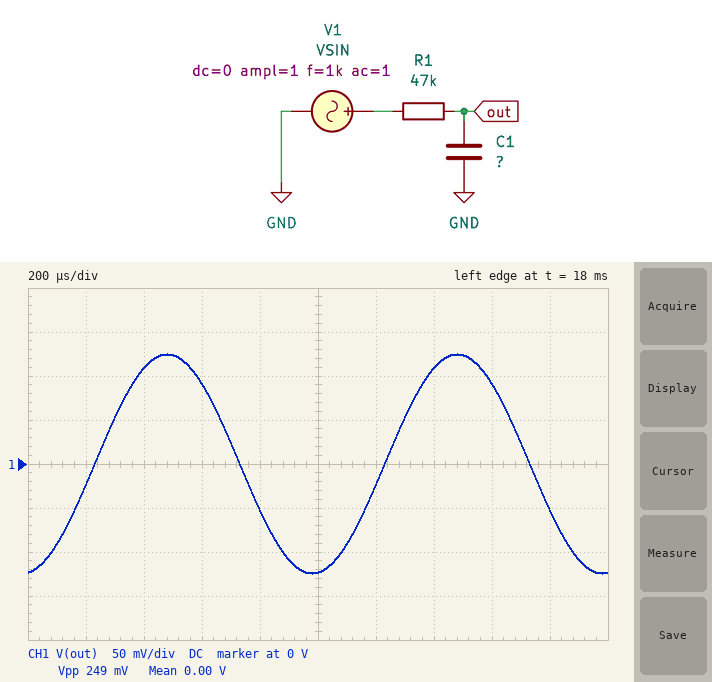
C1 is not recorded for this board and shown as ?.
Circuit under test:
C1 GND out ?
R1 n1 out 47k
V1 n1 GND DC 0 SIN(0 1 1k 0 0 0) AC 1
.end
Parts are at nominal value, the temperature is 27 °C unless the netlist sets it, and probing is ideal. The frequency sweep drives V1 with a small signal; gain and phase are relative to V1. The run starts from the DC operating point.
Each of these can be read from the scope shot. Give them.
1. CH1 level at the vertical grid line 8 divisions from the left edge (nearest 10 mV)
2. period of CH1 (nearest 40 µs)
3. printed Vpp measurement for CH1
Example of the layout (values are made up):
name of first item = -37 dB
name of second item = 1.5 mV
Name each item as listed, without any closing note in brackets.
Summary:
CH1 level at the vertical grid line 8 divisions from the left edge = 90 mV
period of CH1 = 1.00 ms
printed Vpp measurement for CH1 = 249 mV
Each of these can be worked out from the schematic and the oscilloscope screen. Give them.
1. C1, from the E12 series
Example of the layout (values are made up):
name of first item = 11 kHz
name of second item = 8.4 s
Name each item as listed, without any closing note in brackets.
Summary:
C1, from the E12 series = 27 nF
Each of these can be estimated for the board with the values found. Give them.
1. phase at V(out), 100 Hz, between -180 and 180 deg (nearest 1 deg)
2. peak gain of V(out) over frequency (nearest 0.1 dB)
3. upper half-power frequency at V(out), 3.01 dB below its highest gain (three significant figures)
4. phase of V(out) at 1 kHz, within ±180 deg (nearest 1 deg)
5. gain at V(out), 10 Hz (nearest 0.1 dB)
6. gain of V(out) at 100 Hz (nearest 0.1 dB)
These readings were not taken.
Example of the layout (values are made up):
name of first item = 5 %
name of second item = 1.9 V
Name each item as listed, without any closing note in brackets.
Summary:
phase at V(out), 100 Hz, between -180 and 180 deg = -39 deg
peak gain of V(out) over frequency = 0 dB
upper half-power frequency at V(out), 3.01 dB below its highest gain = 125 Hz
phase of V(out) at 1 kHz, within ±180 deg = -83 deg
gain at V(out), 10 Hz = 0 dB
gain of V(out) at 100 Hz = -2.1 dB
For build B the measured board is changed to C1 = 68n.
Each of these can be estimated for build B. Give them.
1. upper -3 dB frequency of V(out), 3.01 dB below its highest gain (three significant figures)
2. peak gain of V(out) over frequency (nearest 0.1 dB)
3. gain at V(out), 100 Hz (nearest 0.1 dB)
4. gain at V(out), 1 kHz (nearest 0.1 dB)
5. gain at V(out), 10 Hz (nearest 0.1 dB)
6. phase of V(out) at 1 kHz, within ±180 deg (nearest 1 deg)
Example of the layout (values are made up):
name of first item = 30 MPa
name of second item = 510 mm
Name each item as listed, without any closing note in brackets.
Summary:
upper -3 dB frequency of V(out), 3.01 dB below its highest gain = 49.8 Hz
peak gain of V(out) over frequency = 0 dB
gain at V(out), 100 Hz = -7.0 dB
gain at V(out), 1 kHz = -26.1 dB
gain at V(out), 10 Hz = -0.2 dB
phase of V(out) at 1 kHz, within ±180 deg = -87 deg
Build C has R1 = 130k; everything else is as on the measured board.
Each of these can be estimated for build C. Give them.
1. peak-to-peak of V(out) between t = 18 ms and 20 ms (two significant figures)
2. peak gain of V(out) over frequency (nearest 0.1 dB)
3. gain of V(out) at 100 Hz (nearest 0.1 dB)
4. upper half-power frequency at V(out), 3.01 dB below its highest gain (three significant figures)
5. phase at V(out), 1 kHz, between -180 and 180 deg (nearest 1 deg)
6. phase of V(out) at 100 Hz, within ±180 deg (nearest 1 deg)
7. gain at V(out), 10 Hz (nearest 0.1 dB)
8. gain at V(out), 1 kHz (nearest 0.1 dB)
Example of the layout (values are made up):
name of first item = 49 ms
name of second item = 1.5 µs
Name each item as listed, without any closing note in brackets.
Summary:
peak-to-peak of V(out) between t = 18 ms and 20 ms = 91 mV
peak gain of V(out) over frequency = 0 dB
gain of V(out) at 100 Hz = -7.7 dB
upper half-power frequency at V(out), 3.01 dB below its highest gain = 45.3 Hz
phase at V(out), 1 kHz, between -180 and 180 deg = -87 deg
phase of V(out) at 100 Hz, within ±180 deg = -66 deg
gain at V(out), 10 Hz = -0.2 dB
gain at V(out), 1 kHz = -26.9 dB
